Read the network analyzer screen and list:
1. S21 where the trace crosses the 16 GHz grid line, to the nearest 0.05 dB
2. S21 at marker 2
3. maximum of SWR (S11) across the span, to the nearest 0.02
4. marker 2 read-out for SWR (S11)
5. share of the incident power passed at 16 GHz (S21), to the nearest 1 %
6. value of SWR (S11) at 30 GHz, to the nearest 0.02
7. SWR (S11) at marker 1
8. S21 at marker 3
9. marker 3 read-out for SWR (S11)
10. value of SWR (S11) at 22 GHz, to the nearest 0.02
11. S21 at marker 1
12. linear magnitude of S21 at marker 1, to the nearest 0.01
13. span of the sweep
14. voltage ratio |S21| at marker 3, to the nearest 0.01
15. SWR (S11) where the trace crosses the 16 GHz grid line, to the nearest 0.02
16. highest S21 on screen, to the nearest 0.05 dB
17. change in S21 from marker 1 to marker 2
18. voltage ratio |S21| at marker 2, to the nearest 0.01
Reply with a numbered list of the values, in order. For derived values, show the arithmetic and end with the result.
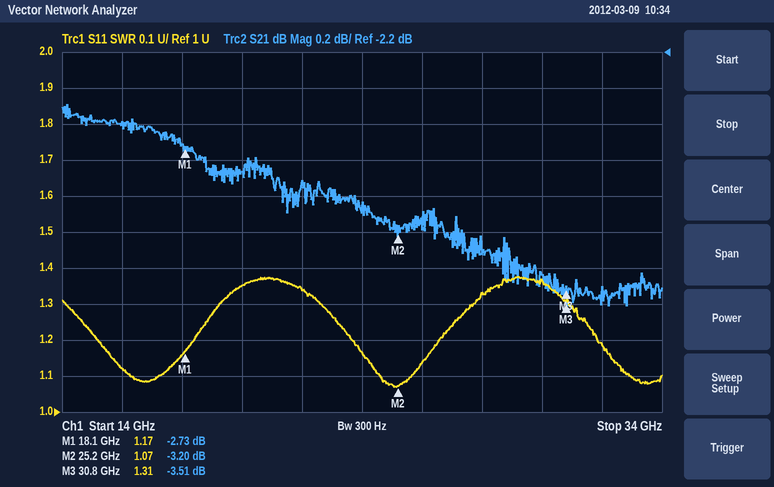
1. -2.60 dB
2. -3.20 dB
3. 1.38
4. 1.07
5. 10^(-2.6/10) ≈ 55 %
6. 1.36
7. 1.17
8. -3.51 dB
9. 1.31
10. 1.34
11. -2.73 dB
12. 10^(-2.73/20) ≈ 0.73
13. 20 GHz
14. 10^(-3.51/20) ≈ 0.67
15. 1.12
16. -2.50 dB
17. -3.2 − (-2.73) = -0.47 dB
18. 10^(-3.2/20) ≈ 0.69
